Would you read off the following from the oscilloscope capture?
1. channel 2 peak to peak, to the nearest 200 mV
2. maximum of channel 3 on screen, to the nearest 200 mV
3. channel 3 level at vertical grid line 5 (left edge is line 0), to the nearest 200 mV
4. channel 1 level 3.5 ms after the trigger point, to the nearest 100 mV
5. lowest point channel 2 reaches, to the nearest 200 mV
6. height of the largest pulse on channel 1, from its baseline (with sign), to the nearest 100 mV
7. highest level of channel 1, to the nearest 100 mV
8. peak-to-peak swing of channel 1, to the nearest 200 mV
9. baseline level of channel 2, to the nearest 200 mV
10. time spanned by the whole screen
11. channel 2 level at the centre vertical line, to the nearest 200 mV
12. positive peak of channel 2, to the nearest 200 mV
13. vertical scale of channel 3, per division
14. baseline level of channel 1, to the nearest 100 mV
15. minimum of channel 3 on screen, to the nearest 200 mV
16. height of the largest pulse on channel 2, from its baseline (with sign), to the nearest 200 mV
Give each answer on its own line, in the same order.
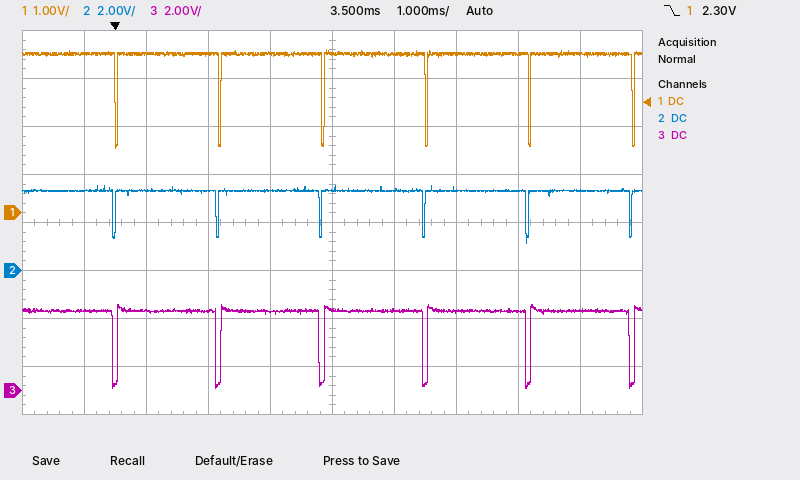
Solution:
2.4 V
3.6 V
3.4 V
3.3 V
1.2 V
-2.0 V
3.4 V
2.0 V
3.4 V
10 ms
3.4 V
3.6 V
2 V
3.3 V
0.0 V
-2.2 V
